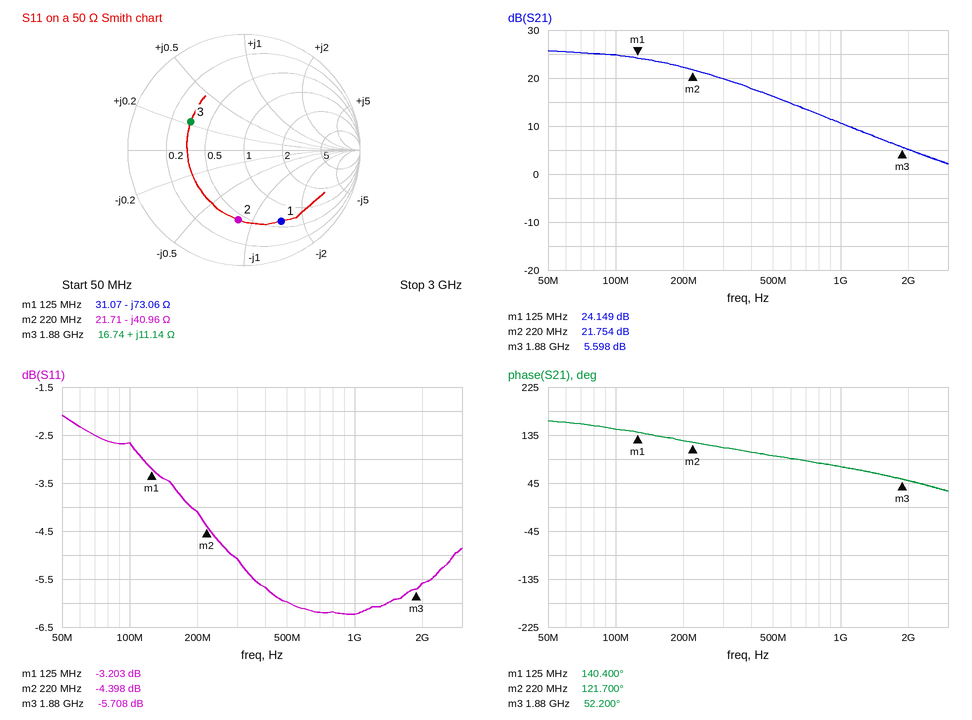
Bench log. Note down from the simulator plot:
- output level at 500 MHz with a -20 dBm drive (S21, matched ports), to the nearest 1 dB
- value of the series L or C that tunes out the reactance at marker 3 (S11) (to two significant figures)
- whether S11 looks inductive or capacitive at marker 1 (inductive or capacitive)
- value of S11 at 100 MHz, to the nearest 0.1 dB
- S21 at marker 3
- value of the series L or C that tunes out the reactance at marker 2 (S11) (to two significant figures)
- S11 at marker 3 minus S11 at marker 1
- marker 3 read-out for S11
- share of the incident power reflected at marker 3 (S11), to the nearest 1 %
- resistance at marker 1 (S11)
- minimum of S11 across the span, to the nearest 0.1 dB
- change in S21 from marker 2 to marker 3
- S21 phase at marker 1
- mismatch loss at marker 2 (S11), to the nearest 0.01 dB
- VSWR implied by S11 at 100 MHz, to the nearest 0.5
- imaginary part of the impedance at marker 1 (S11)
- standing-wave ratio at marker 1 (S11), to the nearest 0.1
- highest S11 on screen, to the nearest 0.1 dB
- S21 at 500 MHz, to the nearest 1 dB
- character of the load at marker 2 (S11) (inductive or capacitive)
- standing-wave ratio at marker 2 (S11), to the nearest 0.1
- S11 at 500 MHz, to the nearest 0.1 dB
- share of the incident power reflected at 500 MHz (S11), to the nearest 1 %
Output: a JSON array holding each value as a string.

["-4 dBm", "7.6 pF", "capacitive", "-2.7 dB", "5.598 dB", "30 nH", "-2.505 dB", "-5.708 dB", "27 %", "31.07 Ω", "-6.2 dB", "-16.156 dB", "140.400°", "1.96 dB", "6.5", "-73.06 Ω", "5.5", "-2.1 dB", "16 dB", "capacitive", "4.0", "-6.0 dB", "25 %"]
